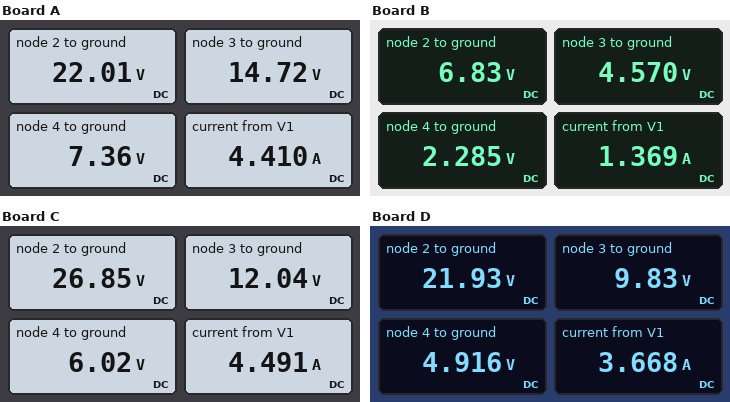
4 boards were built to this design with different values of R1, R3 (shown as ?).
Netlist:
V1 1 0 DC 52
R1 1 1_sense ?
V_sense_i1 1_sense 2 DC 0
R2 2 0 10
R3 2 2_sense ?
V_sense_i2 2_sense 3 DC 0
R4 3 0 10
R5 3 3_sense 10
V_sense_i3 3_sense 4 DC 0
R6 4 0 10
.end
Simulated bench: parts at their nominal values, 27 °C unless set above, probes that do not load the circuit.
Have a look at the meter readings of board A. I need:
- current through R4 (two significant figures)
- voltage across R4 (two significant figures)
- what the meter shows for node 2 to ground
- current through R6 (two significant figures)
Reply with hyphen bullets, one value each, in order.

- 1.5 A
- 15 V
- 22.01 V
- 740 mA
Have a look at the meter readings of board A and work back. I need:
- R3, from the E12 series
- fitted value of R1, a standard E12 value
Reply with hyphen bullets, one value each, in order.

- 3.3 Ω
- 6.8 Ω
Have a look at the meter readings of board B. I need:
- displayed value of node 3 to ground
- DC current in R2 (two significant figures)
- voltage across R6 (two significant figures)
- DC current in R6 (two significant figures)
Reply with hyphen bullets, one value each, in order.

- 4.570 V
- 680 mA
- 2.3 V
- 230 mA
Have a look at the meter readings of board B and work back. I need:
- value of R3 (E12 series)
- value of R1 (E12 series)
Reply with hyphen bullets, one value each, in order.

- 3.3 Ω
- 33 Ω
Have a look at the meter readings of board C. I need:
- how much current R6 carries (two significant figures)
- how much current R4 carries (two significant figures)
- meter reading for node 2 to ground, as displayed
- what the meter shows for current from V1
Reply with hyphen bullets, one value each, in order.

- 600 mA
- 1.2 A
- 26.85 V
- 4.491 A
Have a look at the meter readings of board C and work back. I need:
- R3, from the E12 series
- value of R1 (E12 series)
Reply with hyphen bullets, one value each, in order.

- 8.2 Ω
- 5.6 Ω
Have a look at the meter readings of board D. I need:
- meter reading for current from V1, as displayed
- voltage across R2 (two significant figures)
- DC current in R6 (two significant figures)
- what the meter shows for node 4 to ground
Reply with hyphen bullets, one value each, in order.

- 3.668 A
- 22 V
- 490 mA
- 4.916 V
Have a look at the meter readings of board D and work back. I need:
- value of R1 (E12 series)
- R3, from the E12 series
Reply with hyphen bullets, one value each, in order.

- 8.2 Ω
- 8.2 Ω
